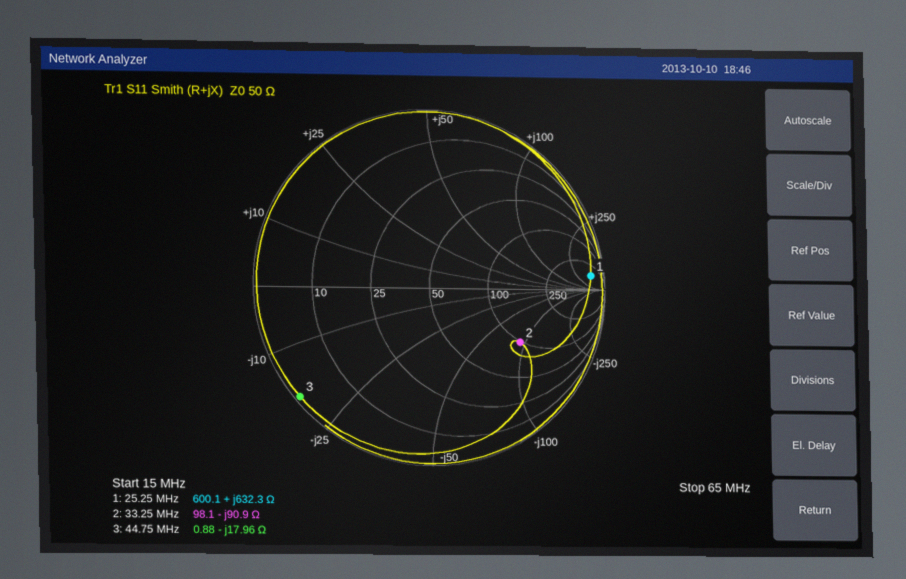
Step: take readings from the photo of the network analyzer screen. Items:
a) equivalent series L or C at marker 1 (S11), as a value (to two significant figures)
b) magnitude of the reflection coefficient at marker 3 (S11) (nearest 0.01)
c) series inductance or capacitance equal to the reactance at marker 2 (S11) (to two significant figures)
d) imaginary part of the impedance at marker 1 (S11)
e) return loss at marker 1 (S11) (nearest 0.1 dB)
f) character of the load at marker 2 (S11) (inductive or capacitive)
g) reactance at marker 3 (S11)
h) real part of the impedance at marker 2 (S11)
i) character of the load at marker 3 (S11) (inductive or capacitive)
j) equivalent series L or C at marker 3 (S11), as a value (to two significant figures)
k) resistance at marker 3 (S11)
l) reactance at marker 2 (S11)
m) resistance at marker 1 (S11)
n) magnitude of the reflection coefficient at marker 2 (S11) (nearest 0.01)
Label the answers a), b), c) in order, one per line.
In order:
a) 4.0 µH
b) 0.97
c) 53 pF
d) +632.3 Ω
e) 0.7 dB
f) capacitive
g) -17.96 Ω
h) 98.1 Ω
i) capacitive
j) 200 pF
k) 0.88 Ω
l) -90.9 Ω
m) 600.1 Ω
n) 0.59
